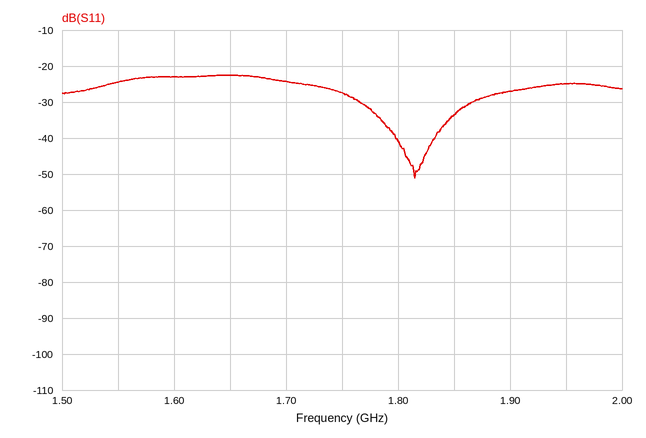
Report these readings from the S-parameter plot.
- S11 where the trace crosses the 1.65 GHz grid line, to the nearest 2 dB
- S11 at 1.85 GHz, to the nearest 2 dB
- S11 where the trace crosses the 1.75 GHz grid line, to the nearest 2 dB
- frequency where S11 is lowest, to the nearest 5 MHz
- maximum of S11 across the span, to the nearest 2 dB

-22 dB
-34 dB
-28 dB
1.815 GHz
-22 dB
